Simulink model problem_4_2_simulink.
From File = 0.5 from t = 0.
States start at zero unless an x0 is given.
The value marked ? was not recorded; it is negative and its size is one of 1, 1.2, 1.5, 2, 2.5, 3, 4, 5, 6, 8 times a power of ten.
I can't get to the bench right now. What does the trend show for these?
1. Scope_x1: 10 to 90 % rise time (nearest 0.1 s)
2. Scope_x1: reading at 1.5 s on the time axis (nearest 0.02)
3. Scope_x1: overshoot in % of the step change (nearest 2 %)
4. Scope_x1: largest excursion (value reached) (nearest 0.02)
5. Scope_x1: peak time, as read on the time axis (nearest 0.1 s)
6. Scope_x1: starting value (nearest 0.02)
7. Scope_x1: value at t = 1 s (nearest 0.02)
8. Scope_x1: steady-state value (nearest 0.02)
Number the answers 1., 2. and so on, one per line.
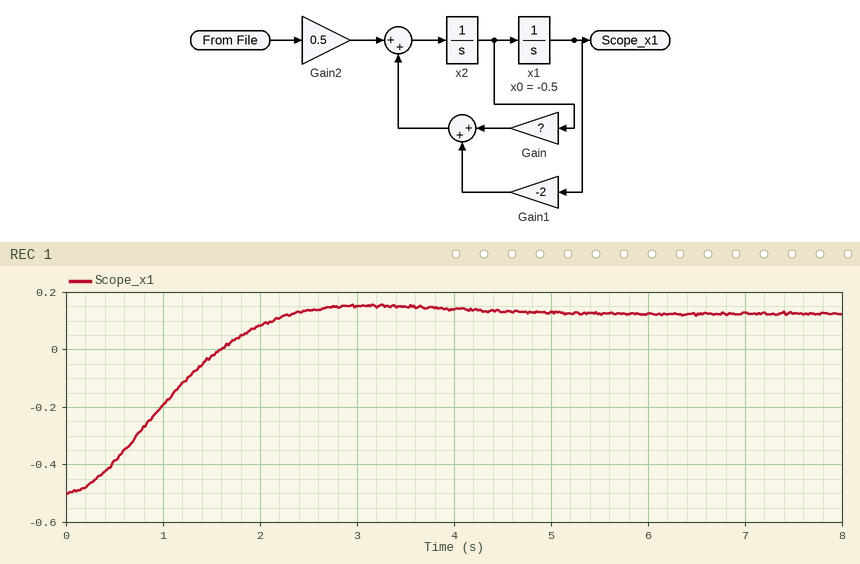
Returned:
1. 1.5 s
2. -0.02
3. 4 %
4. 0.16
5. 3.1 s
6. -0.50
7. -0.20
8. 0.12
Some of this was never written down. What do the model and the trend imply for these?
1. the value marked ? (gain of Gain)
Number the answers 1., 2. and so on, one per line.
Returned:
1. -2
